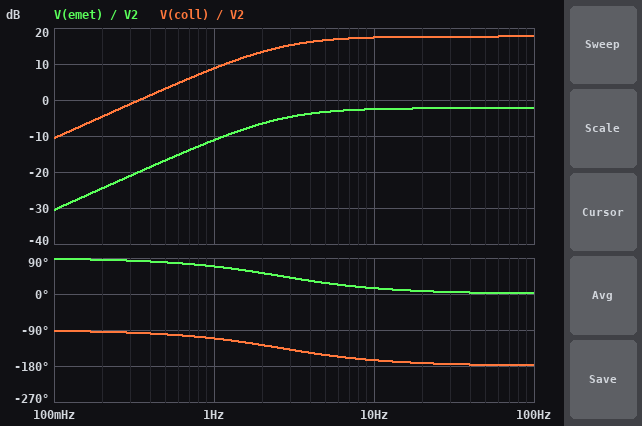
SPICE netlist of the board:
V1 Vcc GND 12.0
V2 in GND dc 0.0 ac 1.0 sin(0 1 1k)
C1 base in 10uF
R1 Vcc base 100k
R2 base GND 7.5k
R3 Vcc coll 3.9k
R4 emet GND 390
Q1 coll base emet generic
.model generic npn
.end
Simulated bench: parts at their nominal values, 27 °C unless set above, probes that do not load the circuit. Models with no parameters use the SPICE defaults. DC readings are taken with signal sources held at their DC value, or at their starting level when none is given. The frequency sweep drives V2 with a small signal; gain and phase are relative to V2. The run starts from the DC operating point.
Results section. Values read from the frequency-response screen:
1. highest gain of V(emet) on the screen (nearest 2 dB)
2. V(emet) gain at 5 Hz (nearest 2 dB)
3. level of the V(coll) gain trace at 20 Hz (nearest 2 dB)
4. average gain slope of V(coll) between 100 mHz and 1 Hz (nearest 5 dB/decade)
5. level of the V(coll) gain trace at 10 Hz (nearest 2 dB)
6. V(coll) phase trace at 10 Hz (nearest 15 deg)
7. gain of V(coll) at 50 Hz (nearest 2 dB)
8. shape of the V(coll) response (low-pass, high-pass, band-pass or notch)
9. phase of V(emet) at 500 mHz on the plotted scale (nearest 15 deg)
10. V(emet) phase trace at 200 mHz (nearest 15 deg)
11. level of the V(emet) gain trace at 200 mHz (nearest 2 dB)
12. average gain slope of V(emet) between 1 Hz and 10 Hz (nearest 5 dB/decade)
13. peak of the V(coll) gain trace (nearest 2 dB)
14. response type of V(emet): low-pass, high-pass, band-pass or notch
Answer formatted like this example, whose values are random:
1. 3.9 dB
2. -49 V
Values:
1. -2 dB
2. -4 dB
3. 18 dB
4. 20 dB/decade
5. 18 dB
6. -165 deg
7. 18 dB
8. high-pass
9. 75 deg
10. 90 deg
11. -24 dB
12. 10 dB/decade
13. 18 dB
14. high-pass
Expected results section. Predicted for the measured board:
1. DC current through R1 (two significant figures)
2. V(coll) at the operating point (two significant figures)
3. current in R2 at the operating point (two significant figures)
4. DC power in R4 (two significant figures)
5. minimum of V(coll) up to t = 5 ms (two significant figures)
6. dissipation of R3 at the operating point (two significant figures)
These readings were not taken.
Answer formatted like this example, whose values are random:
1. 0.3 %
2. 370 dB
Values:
1. 110 µA
2. 11 V
3. 110 µA
4. 19 µW
5. 1.9 V
6. 190 µW
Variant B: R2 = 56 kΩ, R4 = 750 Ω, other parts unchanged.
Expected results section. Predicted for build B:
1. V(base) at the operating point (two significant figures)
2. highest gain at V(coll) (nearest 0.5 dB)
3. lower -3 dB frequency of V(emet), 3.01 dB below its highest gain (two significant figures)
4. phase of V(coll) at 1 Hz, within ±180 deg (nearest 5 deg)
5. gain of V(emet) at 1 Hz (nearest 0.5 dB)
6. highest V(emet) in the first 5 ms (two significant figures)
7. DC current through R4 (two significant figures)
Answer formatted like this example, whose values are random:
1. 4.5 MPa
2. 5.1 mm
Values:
1. 2.7 V
2. -4.0 dB
3. 19 Hz
4. -95 deg
5. -25.5 dB
6. 2.9 V
7. 2.6 mA
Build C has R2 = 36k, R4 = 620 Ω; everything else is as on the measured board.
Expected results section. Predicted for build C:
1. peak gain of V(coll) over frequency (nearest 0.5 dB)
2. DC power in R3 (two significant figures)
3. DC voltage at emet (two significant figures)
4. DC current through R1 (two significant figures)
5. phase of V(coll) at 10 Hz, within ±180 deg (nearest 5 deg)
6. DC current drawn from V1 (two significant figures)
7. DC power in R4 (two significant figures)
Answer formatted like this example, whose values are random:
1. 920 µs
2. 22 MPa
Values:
1. 13.0 dB
2. 27 mW
3. 1.6 V
4. 96 µA
5. -145 deg
6. 2.7 mA
7. 4.3 mW
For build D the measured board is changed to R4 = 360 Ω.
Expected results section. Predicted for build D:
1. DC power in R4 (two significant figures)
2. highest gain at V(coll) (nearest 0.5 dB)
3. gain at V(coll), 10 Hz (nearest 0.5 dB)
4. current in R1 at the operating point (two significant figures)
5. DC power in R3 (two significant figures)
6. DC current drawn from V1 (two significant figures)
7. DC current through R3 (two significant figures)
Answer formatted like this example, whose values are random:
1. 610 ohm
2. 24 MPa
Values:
1. 20 µW
2. 18.5 dB
3. 18.0 dB
4. 110 µA
5. 210 µW
6. 340 µA
7. 230 µA
